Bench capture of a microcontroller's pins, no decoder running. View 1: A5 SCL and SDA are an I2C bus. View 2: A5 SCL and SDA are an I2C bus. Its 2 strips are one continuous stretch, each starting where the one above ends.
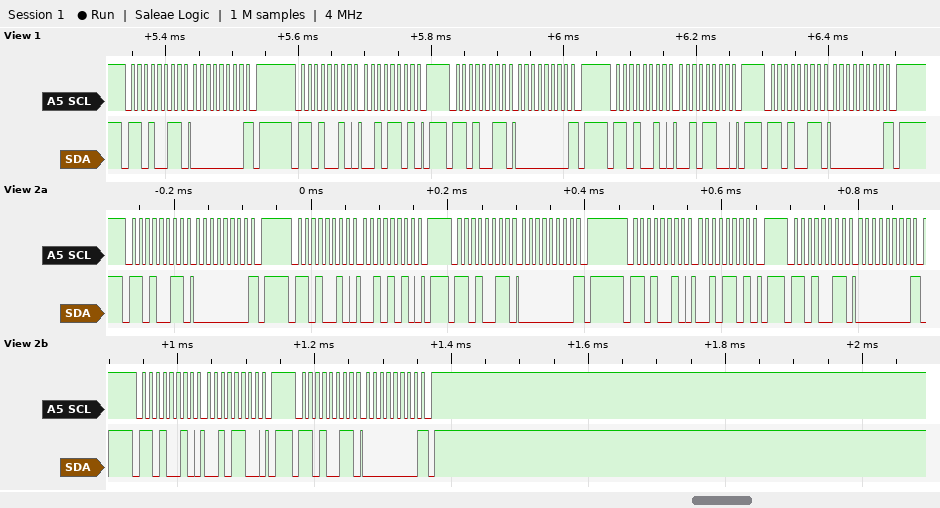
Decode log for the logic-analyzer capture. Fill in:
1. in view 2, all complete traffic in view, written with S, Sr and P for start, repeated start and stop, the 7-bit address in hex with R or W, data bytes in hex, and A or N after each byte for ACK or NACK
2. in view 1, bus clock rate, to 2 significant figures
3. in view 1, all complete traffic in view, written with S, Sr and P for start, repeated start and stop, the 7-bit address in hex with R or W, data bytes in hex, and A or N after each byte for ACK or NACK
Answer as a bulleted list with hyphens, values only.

- S 69R A 00 N P S 69W A 2A A P S 69R A 00 N P S 69W A 2D A P S 69R A 00 N P S 69W A 2C A P S 69R A 00 N P
- 100 kHz
- S 69R A 00 N P S 69W A 2D A P S 69R A 00 N P S 69W A 2C A P S 69R A 00 N P
